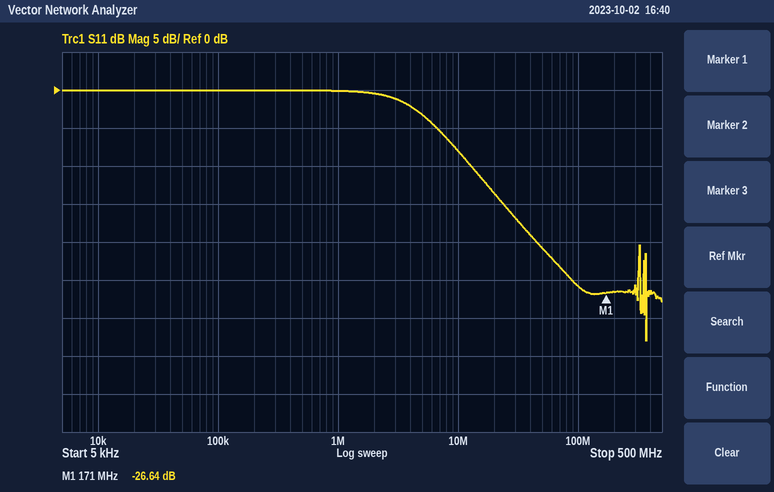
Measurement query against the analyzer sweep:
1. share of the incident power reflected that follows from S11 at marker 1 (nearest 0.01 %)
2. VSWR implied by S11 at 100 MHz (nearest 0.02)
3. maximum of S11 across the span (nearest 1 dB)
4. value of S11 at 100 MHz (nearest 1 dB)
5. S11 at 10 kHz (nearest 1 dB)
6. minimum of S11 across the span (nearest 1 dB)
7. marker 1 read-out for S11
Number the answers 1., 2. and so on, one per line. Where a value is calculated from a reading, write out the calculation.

1. 10^(-26.64/10) ≈ 0.22 %
2. |Γ| = 10^(-26/20) = 0.0501; VSWR = (1 + 0.0501)/(1 − 0.0501) ≈ 1.11, so 1.10 to the nearest 0.02
3. 0 dB
4. -26 dB
5. 0 dB
6. -33 dB
7. -26.64 dB
